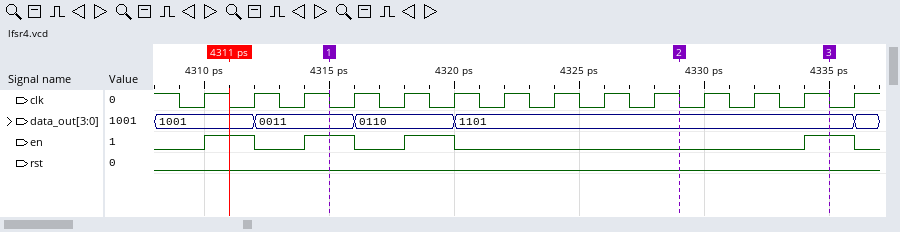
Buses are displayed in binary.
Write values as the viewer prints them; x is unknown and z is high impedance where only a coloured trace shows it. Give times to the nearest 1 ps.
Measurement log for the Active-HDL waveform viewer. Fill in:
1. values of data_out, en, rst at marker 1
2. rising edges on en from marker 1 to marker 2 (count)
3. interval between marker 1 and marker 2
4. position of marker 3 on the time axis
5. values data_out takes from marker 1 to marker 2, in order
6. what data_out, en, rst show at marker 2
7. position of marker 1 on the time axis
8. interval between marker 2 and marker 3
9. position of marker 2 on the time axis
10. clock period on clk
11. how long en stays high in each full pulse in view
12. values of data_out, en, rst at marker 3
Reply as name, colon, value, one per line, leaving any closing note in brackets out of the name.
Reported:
values of data_out, en, rst at marker 1: data_out=0011, en=1, rst=0
rising edges on en from marker 1 to marker 2: 1
interval between marker 1 and marker 2: 14 ps
position of marker 3 on the time axis: 4335 ps
values data_out takes from marker 1 to marker 2, in order: 0011, 0110, 1101
what data_out, en, rst show at marker 2: data_out=1101, en=0, rst=0
position of marker 1 on the time axis: 4315 ps
interval between marker 2 and marker 3: 6 ps
position of marker 2 on the time axis: 4329 ps
clock period on clk: 2 ps
how long en stays high in each full pulse in view: 2 ps, 2 ps, 2 ps, 2 ps
values of data_out, en, rst at marker 3: data_out=1101, en=1, rst=0
